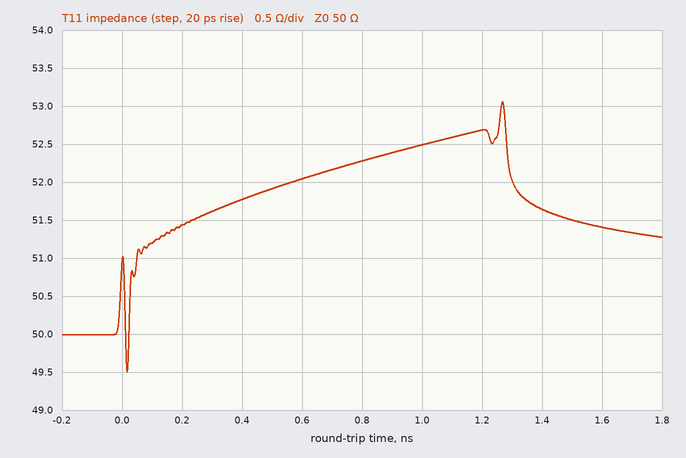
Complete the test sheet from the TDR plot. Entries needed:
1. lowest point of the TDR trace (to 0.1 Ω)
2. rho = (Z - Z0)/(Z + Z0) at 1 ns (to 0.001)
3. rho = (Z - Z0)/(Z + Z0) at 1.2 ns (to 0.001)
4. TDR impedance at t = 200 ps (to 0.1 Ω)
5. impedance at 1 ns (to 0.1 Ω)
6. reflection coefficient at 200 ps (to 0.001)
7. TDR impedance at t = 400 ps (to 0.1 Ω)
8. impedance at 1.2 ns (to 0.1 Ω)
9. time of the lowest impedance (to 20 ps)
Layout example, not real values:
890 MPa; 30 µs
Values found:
49.5 Ω; +0.024; +0.026; 51.4 Ω; 52.5 Ω; +0.014; 51.8 Ω; 52.7 Ω; 20 ps
